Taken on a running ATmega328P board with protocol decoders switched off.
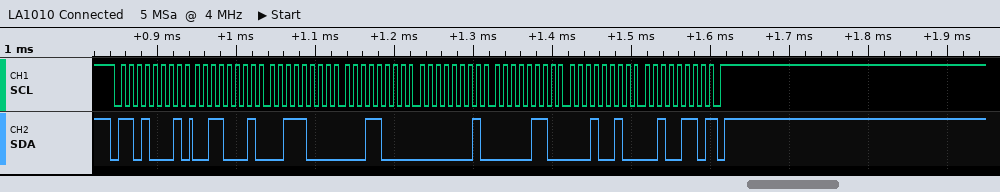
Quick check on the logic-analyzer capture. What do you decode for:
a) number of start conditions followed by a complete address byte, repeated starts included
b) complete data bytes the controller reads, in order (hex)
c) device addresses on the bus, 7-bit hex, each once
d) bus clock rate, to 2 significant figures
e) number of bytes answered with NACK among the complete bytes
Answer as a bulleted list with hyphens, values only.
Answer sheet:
- 1
- 31 38 18 01 06 12 26
- 0x68
- 100 kHz
- 1
